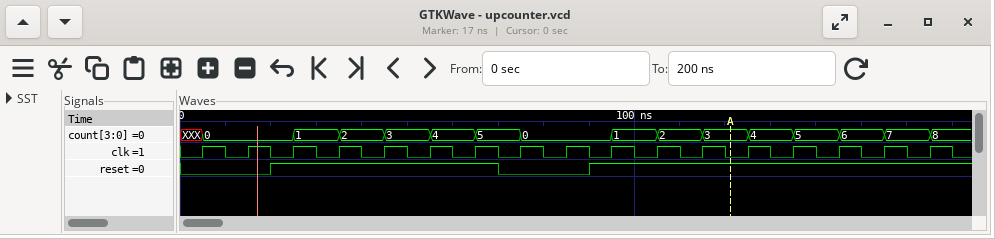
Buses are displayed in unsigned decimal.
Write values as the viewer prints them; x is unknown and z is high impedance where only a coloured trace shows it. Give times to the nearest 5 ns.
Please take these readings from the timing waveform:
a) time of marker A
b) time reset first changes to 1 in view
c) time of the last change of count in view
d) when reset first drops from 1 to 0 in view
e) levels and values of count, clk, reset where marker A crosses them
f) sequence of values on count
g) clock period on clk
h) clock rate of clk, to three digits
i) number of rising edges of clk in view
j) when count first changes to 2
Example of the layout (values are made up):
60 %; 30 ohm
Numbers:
120 ns; 20 ns; 165 ns; 70 ns; count=3, clk=0, reset=1; XXX, 0, 1, 2, 3, 4, 5, 0, 1, 2, 3, 4, 5, 6, 7, 8; 10 ns; 100 MHz; 17; 35 ns
